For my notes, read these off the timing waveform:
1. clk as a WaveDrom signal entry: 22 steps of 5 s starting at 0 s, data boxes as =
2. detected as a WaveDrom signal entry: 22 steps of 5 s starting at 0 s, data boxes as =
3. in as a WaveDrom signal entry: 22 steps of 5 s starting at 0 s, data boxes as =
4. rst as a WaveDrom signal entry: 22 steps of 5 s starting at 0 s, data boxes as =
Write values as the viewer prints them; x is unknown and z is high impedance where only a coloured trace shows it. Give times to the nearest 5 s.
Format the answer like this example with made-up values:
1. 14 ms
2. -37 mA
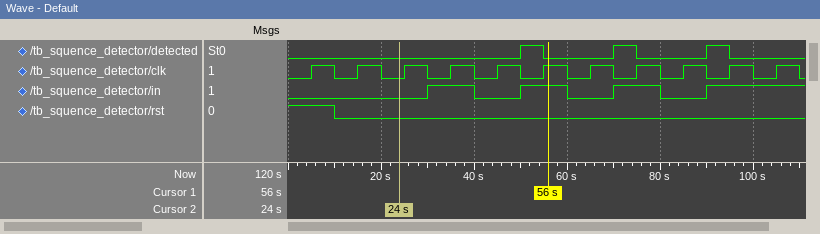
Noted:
1. {name: 'clk', wave: '0101010101010101010101'}
2. {name: 'detected', wave: '0.........10..10..10..'}
3. {name: 'in', wave: '0.....1.0.1.0.1.0.1...'}
4. {name: 'rst', wave: '1.0...................'}
